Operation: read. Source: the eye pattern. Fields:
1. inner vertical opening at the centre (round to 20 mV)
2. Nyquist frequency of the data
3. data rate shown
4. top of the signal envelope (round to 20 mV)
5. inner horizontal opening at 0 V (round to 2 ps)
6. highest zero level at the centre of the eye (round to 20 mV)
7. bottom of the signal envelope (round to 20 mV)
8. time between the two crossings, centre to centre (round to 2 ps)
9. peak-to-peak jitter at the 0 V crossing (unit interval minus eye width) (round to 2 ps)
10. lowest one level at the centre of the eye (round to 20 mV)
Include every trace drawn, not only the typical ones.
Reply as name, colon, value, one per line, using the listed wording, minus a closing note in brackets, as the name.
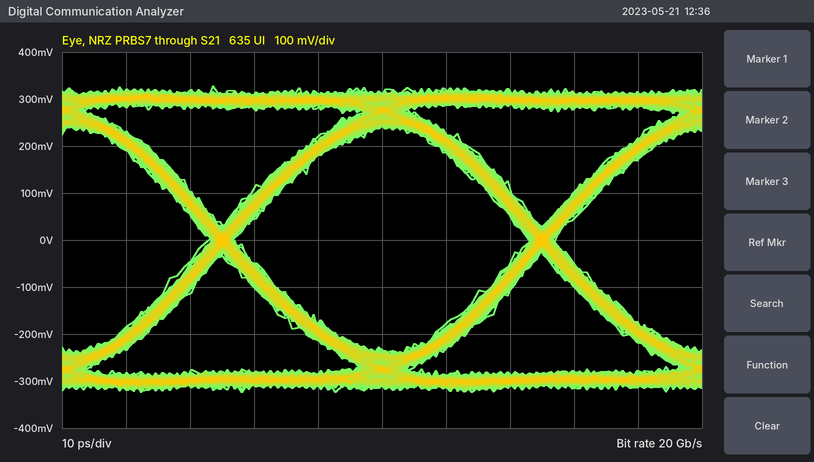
inner vertical opening at the centre: 480 mV
Nyquist frequency of the data: 10 GHz
data rate shown: 20 Gb/s
top of the signal envelope: 320 mV
inner horizontal opening at 0 V: 46 ps
highest zero level at the centre of the eye: -240 mV
bottom of the signal envelope: -320 mV
time between the two crossings, centre to centre: 50 ps
peak-to-peak jitter at the 0 V crossing (unit interval minus eye width): 4 ps
lowest one level at the centre of the eye: 240 mV
